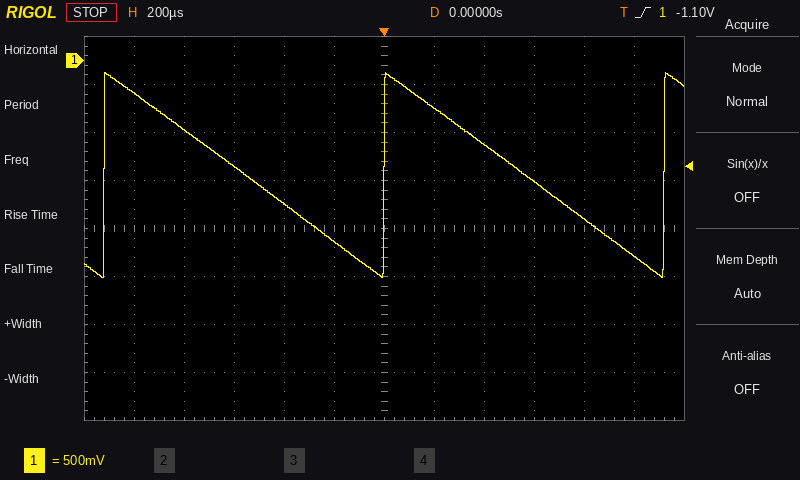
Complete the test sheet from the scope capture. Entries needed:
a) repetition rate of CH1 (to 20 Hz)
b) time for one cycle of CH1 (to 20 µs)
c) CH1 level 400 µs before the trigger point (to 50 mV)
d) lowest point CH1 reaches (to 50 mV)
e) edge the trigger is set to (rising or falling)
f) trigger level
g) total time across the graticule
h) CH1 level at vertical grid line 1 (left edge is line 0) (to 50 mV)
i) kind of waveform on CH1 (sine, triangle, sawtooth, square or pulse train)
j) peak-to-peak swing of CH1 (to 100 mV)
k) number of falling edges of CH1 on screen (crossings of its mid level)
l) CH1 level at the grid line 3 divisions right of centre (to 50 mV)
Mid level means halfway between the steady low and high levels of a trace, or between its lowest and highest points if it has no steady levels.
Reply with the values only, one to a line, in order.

900 Hz
1.12 ms
-1.50 V
-2.25 V
rising
-1.10 V
2.4 ms
-350 mV
sawtooth
2.10 V
2
-1.25 V
